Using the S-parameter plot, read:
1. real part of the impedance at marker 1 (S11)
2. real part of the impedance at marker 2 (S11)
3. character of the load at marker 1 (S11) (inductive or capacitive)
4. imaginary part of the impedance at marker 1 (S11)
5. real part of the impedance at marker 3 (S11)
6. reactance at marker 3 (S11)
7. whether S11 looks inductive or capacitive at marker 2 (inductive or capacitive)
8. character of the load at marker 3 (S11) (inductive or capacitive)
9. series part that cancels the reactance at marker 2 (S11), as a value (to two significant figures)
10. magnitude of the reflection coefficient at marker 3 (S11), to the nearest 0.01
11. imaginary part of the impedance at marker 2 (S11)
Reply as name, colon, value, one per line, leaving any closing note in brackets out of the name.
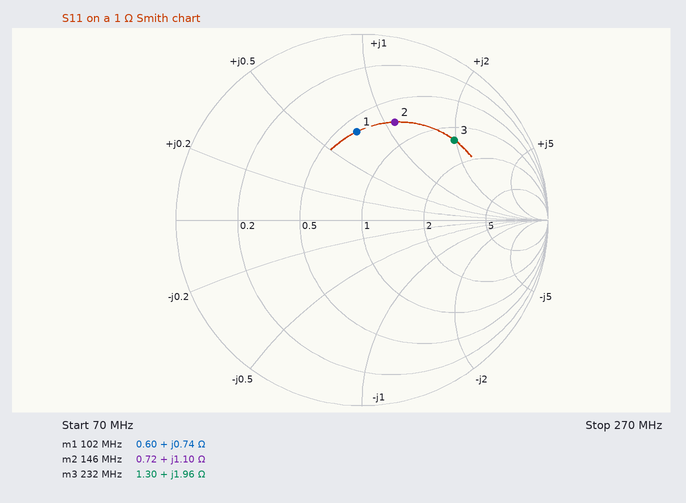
real part of the impedance at marker 1: 0.60 Ω
real part of the impedance at marker 2: 0.72 Ω
character of the load at marker 1 (S11): inductive
imaginary part of the impedance at marker 1: +0.74 Ω
real part of the impedance at marker 3: 1.30 Ω
reactance at marker 3: +1.96 Ω
whether S11 looks inductive or capacitive at marker 2: inductive
character of the load at marker 3 (S11): inductive
series part that cancels the reactance at marker 2 (S11), as a value: 990 pF
magnitude of the reflection coefficient at marker 3 (S11), to the nearest 0.01: 0.66
imaginary part of the impedance at marker 2: +1.10 Ω
